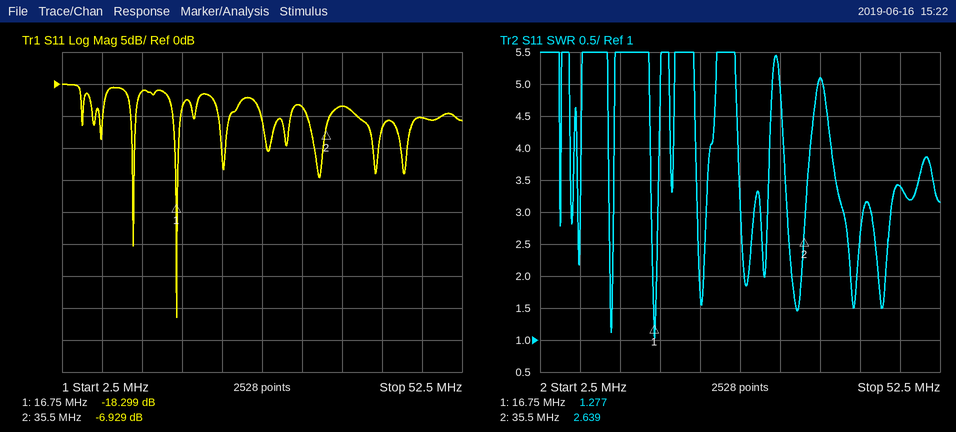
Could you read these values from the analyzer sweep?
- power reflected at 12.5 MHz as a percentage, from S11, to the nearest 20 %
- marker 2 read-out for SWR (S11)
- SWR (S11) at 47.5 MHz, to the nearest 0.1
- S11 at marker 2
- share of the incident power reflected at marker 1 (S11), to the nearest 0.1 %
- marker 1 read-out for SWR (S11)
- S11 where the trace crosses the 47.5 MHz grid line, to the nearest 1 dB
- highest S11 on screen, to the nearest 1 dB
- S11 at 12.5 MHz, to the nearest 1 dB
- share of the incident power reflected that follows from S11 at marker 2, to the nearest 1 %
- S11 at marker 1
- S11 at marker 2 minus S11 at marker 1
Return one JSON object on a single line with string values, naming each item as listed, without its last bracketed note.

{"power reflected at 12.5 MHz as a percentage, from S11, to the nearest 20 %": "80 %", "marker 2 read-out for SWR": "2.639", "SWR (S11) at 47.5 MHz, to the nearest 0.1": "3.4", "S11 at marker 2": "-6.929 dB", "share of the incident power reflected at marker 1 (S11), to the nearest 0.1 %": "1.5 %", "marker 1 read-out for SWR": "1.277", "S11 where the trace crosses the 47.5 MHz grid line, to the nearest 1 dB": "-5 dB", "highest S11 on screen, to the nearest 1 dB": "0 dB", "S11 at 12.5 MHz, to the nearest 1 dB": "-1 dB", "share of the incident power reflected that follows from S11 at marker 2, to the nearest 1 %": "20 %", "S11 at marker 1": "-18.299 dB", "S11 at marker 2 minus S11 at marker 1": "11.370 dB"}
